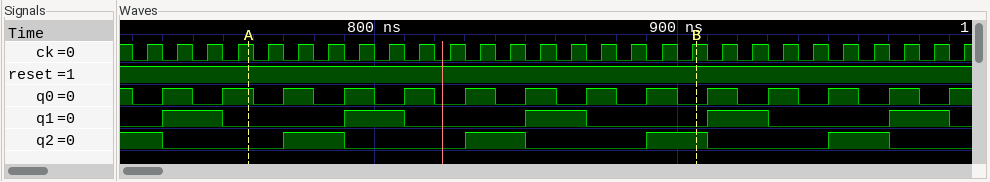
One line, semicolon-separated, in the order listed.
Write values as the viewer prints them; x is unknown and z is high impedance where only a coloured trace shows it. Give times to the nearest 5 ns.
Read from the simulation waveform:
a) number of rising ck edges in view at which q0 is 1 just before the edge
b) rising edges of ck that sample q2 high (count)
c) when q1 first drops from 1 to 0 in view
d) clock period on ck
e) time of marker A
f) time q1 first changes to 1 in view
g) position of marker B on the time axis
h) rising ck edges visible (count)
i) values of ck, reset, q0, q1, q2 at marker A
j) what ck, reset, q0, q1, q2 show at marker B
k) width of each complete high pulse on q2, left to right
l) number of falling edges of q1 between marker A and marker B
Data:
14; 9; 750 ns; 10 ns; 760 ns; 730 ns; 905 ns; 28; ck=1, reset=1, q0=1, q1=0, q2=0; ck=1, reset=1, q0=0, q1=0, q2=1; 20 ns, 20 ns, 20 ns, 20 ns; 2
